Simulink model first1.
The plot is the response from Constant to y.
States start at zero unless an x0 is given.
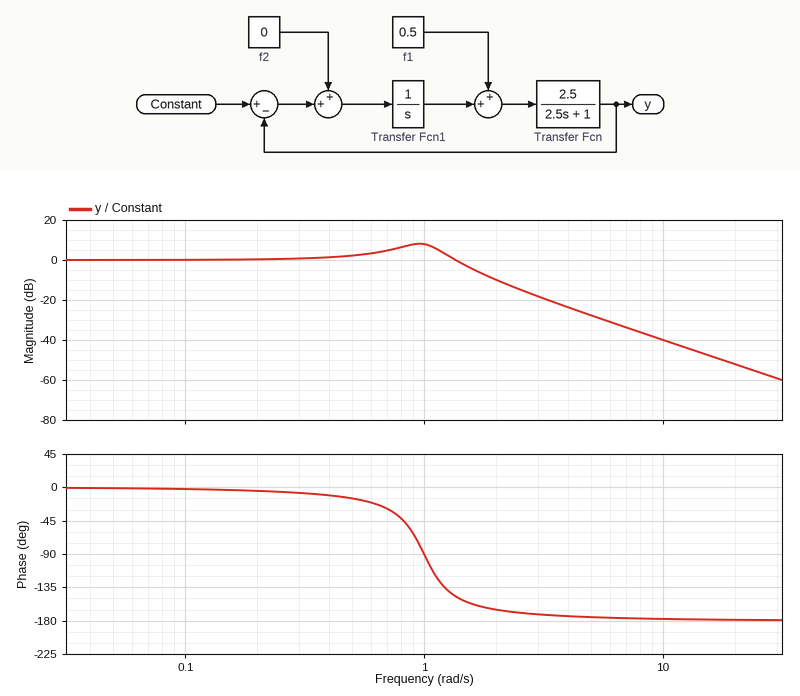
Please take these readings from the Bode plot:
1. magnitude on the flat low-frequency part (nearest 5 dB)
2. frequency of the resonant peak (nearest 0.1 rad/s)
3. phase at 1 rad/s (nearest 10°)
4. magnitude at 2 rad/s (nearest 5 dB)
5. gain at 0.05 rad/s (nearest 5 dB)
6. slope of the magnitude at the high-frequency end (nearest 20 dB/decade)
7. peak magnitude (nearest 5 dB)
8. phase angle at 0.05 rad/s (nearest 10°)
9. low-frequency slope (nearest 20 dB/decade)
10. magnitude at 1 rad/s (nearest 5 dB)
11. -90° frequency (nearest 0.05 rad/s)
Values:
0 dB
1.0 rad/s
-90°
-10 dB
0 dB
-40 dB/decade
10 dB
0°
0 dB/decade
10 dB
1.00 rad/s
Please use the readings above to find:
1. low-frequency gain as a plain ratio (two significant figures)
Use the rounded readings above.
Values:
1.0
